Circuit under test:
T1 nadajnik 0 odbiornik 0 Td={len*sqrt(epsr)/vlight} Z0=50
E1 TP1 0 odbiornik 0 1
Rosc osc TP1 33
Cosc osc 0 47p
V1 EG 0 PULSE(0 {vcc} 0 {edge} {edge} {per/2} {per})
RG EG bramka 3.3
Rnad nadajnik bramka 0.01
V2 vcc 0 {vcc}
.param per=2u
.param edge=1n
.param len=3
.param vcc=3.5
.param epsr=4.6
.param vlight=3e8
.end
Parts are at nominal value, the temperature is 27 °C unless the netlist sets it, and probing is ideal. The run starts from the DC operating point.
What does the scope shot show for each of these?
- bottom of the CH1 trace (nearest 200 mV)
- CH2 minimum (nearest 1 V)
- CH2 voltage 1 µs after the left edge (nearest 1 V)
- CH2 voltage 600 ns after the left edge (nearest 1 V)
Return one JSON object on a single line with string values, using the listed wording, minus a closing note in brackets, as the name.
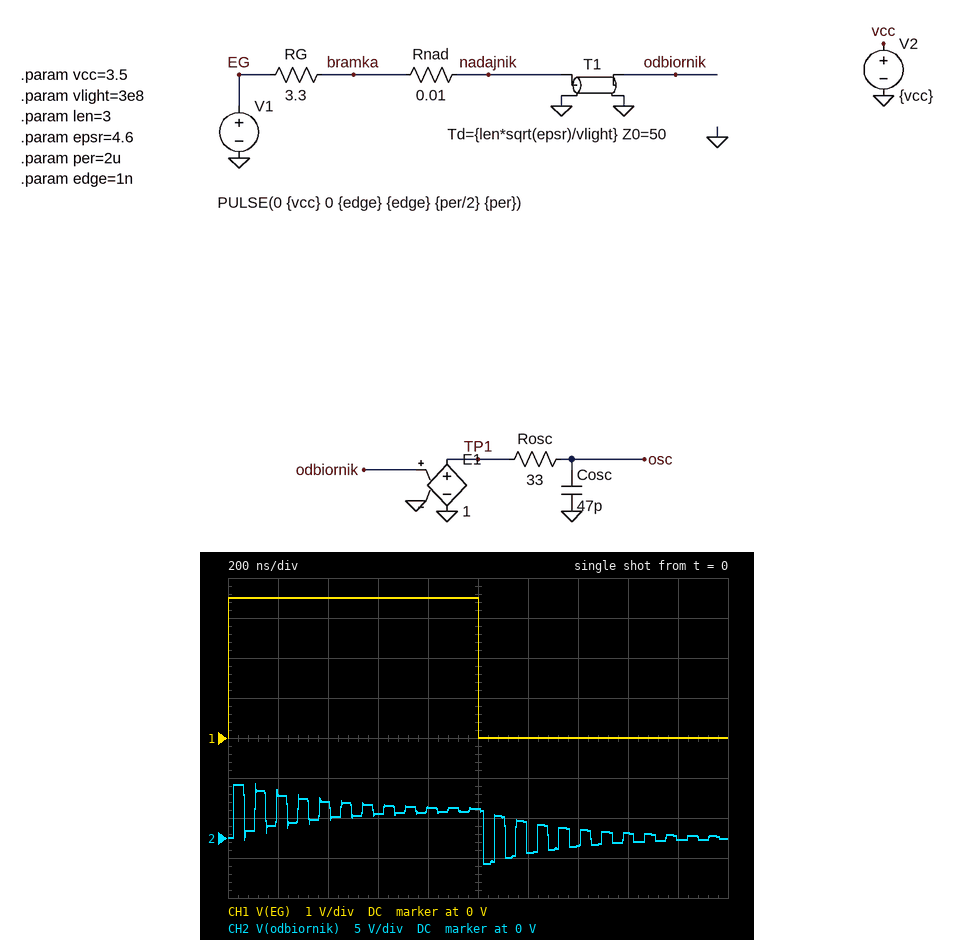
{"bottom of the CH1 trace": "0 V", "CH2 minimum": "-3 V", "CH2 voltage 1 µs after the left edge": "4 V", "CH2 voltage 600 ns after the left edge": "3 V"}
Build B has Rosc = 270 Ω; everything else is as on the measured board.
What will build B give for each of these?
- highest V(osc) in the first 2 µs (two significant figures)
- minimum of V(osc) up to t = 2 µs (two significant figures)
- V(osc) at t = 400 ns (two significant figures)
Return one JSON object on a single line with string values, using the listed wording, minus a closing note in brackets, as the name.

{"highest V(osc) in the first 2 µs": "6.3 V", "minimum of V(osc) up to t = 2 µs": "-2.8 V", "V(osc) at t = 400 ns": "4.4 V"}
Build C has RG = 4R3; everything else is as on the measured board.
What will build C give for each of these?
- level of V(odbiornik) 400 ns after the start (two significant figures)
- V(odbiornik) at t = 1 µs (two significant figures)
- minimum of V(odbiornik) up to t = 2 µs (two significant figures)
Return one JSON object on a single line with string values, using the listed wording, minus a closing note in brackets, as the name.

{"level of V(odbiornik) 400 ns after the start": "4.2 V", "V(odbiornik) at t = 1 µs": "3.6 V", "minimum of V(odbiornik) up to t = 2 µs": "-3.0 V"}
